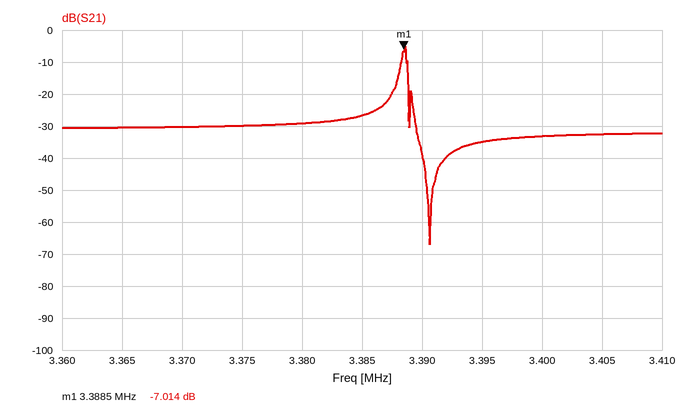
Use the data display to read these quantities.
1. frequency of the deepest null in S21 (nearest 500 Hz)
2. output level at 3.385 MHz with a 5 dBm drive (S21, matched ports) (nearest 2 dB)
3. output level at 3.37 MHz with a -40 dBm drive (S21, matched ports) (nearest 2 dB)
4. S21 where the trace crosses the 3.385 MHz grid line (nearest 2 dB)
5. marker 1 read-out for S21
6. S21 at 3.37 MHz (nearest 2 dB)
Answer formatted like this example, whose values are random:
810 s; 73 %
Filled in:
3.3905 MHz; -22 dBm; -70 dBm; -26 dB; -7.014 dB; -30 dB
